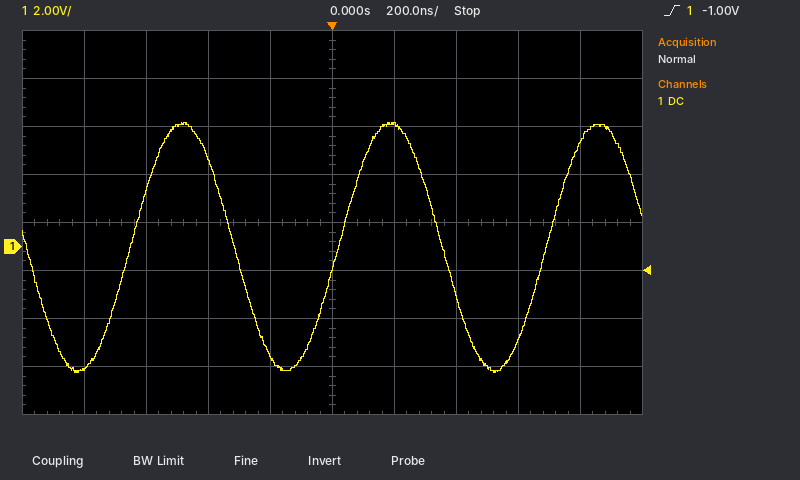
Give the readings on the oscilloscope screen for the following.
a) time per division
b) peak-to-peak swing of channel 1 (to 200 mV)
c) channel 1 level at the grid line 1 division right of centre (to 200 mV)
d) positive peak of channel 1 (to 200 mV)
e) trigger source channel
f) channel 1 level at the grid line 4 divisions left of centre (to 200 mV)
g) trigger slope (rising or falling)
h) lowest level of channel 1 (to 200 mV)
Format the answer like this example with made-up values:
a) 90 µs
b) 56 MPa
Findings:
a) 200 ns
b) 10.4 V
c) 5.0 V
d) 5.2 V
e) channel 1
f) -5.0 V
g) rising
h) -5.2 V
